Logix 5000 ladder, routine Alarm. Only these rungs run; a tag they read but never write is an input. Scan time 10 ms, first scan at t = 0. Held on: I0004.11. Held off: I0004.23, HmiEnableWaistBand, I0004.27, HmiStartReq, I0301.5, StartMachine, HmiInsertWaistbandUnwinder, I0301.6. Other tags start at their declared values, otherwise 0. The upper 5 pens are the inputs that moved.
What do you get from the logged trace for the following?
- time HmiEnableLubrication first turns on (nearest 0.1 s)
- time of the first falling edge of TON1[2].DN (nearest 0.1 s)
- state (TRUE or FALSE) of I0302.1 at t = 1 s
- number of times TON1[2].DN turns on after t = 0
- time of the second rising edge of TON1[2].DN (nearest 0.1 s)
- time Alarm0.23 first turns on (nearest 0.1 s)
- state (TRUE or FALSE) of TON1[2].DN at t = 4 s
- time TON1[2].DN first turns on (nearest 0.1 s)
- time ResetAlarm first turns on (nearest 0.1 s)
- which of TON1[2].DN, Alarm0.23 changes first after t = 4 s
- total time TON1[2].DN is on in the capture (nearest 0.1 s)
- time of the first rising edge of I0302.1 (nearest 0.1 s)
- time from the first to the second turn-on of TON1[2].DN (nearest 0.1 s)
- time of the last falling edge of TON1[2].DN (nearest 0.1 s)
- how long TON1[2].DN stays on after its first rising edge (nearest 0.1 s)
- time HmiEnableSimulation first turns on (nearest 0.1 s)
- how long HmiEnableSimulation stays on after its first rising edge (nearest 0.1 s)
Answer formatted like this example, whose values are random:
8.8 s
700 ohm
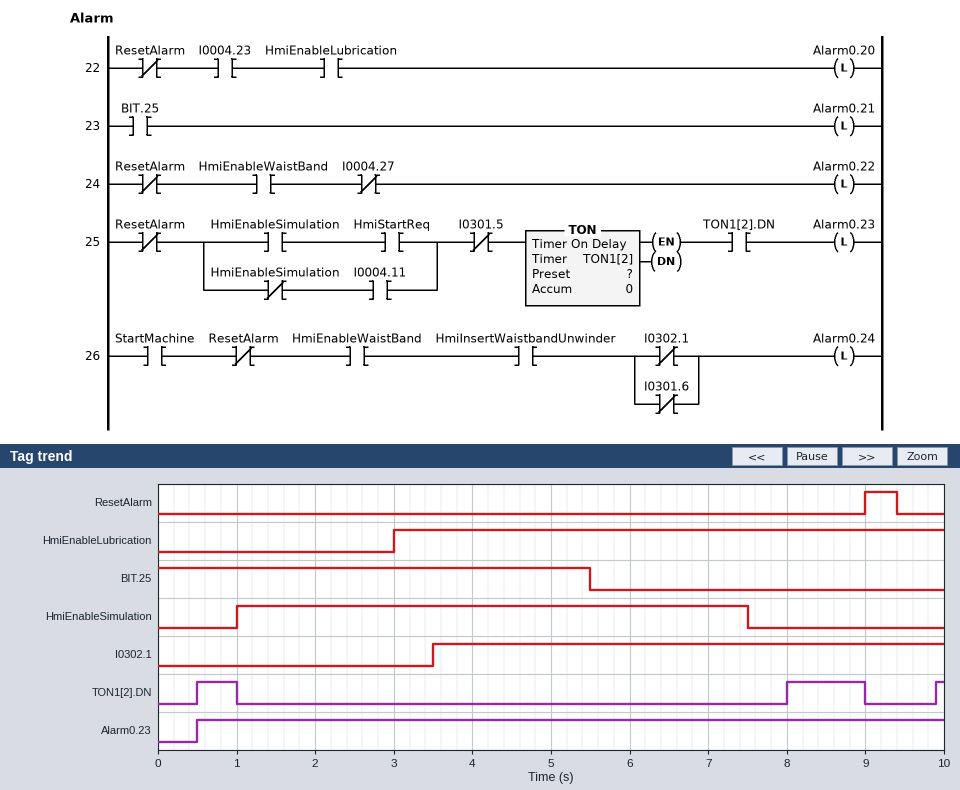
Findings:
3.0 s
1.0 s
FALSE
3
8.0 s
0.5 s
FALSE
0.5 s
9.0 s
TON1[2].DN
1.6 s
3.5 s
7.5 s
9.0 s
0.5 s
1.0 s
6.5 s
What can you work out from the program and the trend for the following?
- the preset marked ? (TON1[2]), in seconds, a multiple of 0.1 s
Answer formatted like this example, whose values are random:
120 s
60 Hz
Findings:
0.5 s
